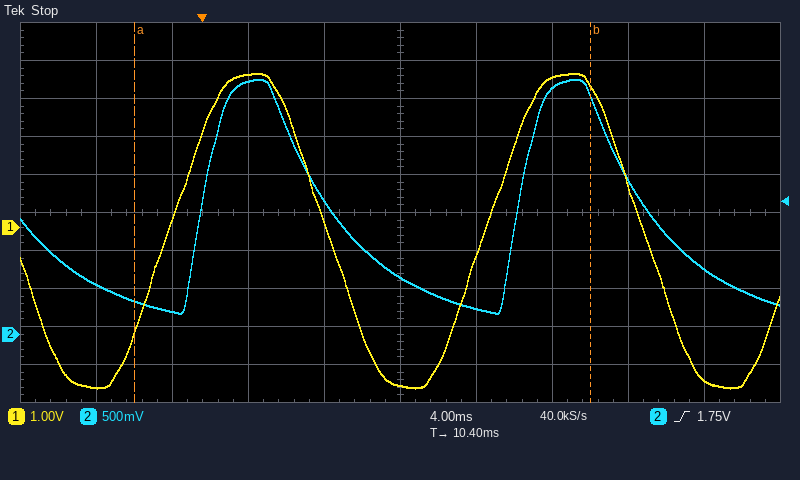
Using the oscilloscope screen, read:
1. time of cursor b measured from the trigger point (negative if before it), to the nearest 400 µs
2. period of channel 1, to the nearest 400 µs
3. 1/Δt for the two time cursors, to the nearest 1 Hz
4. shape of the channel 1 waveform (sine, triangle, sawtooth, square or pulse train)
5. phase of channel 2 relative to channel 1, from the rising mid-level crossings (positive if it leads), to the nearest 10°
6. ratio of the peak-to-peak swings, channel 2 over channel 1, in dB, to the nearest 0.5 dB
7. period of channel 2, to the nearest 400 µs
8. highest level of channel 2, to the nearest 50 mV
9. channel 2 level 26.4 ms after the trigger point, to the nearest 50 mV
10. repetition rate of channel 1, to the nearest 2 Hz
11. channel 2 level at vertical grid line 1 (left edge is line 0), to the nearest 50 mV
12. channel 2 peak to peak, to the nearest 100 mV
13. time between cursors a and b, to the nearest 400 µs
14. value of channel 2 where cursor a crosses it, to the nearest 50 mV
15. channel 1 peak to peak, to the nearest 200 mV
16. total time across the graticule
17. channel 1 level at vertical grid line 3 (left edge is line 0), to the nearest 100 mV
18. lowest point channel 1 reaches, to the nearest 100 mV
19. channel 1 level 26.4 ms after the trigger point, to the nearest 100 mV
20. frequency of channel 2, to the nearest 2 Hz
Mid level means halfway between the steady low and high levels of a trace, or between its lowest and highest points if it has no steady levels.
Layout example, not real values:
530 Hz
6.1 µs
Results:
+20.4 ms
16.8 ms
42 Hz
sine
-40°
-8.5 dB
16.8 ms
3.35 V
850 mV
60 Hz
650 mV
3.10 V
24.0 ms
450 mV
8.2 V
40 ms
4.0 V
-4.2 V
-4.0 V
60 Hz
